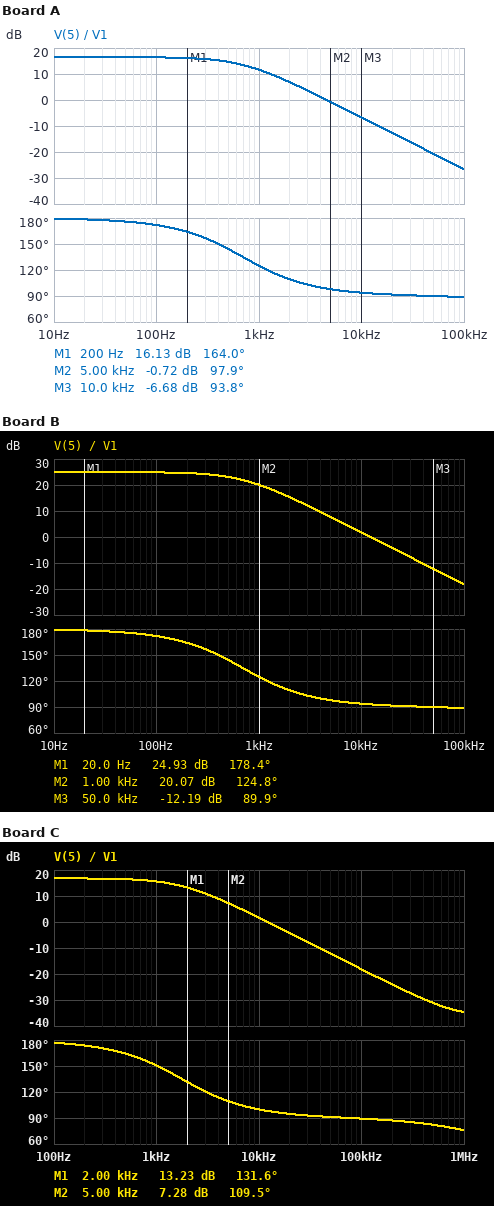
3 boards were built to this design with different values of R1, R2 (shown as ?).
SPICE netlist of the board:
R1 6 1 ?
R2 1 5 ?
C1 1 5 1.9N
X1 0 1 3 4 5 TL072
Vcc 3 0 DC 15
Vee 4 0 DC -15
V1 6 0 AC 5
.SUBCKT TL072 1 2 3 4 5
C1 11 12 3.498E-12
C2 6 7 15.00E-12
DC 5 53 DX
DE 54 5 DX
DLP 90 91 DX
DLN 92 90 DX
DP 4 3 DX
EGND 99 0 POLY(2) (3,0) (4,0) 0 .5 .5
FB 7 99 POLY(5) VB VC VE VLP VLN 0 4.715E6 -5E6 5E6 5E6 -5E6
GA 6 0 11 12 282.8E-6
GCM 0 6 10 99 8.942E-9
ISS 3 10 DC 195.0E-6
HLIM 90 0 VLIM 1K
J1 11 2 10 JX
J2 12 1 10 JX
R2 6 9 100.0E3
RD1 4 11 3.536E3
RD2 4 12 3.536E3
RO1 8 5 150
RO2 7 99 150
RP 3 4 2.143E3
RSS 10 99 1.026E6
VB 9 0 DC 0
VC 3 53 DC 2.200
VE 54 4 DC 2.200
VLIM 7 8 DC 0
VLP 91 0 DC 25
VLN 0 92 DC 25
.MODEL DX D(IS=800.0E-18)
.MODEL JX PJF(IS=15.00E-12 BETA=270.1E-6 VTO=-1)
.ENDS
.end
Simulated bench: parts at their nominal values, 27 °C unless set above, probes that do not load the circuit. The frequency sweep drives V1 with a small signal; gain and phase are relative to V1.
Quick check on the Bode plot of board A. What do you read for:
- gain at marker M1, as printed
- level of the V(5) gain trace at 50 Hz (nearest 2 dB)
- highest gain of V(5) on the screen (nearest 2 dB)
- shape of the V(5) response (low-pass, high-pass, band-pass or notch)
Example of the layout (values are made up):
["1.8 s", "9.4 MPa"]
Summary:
["16.13 dB", "16 dB", "16 dB", "low-pass"]
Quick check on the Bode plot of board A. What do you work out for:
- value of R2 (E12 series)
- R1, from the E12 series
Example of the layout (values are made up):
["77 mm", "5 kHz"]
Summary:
["120 kΩ", "18 kΩ"]
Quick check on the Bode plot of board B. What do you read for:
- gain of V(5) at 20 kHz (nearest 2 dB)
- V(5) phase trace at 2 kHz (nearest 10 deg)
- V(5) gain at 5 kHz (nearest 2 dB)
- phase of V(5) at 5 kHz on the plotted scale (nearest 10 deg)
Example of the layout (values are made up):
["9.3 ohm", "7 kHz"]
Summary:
["-4 dB", "110 deg", "8 dB", "100 deg"]
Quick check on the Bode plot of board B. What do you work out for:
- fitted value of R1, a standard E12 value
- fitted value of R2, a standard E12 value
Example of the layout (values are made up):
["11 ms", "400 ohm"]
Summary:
["6.8 kΩ", "120 kΩ"]
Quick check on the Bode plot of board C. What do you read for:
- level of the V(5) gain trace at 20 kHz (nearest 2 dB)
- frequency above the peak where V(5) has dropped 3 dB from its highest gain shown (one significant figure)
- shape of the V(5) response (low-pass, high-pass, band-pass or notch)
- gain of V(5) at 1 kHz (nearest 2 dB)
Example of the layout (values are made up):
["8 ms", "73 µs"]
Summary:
["-4 dB", "2 kHz", "low-pass", "16 dB"]
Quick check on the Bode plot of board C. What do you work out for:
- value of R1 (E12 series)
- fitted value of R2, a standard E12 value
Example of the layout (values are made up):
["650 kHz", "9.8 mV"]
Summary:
["6.8 kΩ", "47 kΩ"]
